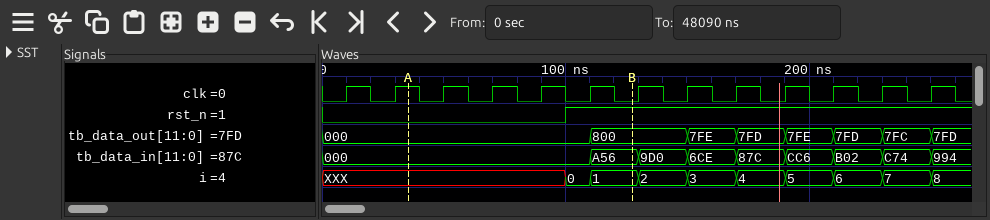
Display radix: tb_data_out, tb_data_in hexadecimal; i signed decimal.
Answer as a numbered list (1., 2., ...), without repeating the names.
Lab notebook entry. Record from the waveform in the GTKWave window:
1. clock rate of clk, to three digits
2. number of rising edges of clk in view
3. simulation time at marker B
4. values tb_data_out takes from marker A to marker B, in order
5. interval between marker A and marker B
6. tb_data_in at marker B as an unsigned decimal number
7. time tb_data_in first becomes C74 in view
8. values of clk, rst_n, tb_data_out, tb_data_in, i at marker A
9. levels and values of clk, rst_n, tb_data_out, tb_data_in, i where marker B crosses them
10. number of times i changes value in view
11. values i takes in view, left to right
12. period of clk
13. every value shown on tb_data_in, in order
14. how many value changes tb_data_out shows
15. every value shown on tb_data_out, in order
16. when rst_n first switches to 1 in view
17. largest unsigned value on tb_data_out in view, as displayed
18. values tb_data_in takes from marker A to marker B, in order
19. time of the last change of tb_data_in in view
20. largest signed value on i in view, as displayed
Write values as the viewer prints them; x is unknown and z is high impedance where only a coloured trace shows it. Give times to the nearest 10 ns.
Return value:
1. 50.0 MHz
2. 13
3. 130 ns
4. 000, 800
5. 90 ns
6. 2646
7. 230 ns
8. clk=1, rst_n=0, tb_data_out=000, tb_data_in=000, i=XXX
9. clk=0, rst_n=1, tb_data_out=800, tb_data_in=A56, i=1
10. 9
11. XXX, 0, 1, 2, 3, 4, 5, 6, 7, 8
12. 20 ns
13. 000, A56, 9D0, 6CE, 87C, CC6, B02, C74, 994
14. 7
15. 000, 800, 7FE, 7FD, 7FE, 7FD, 7FC, 7FD
16. 100 ns
17. 800
18. 000, A56
19. 250 ns
20. 8
